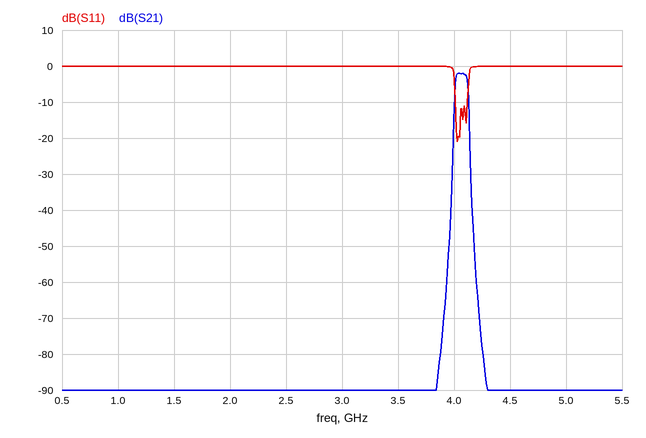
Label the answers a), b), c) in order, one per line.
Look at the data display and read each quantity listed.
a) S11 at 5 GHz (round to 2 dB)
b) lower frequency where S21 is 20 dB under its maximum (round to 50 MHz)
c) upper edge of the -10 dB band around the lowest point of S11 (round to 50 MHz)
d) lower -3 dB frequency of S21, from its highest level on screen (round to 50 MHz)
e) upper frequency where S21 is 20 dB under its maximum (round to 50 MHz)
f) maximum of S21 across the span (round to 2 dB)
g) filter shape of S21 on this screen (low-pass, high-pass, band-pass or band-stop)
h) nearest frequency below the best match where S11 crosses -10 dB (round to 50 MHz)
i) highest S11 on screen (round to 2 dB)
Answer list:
a) 0 dB
b) 4.00 GHz
c) 4.10 GHz
d) 4.00 GHz
e) 4.15 GHz
f) -2 dB
g) band-pass
h) 4.00 GHz
i) 0 dB
